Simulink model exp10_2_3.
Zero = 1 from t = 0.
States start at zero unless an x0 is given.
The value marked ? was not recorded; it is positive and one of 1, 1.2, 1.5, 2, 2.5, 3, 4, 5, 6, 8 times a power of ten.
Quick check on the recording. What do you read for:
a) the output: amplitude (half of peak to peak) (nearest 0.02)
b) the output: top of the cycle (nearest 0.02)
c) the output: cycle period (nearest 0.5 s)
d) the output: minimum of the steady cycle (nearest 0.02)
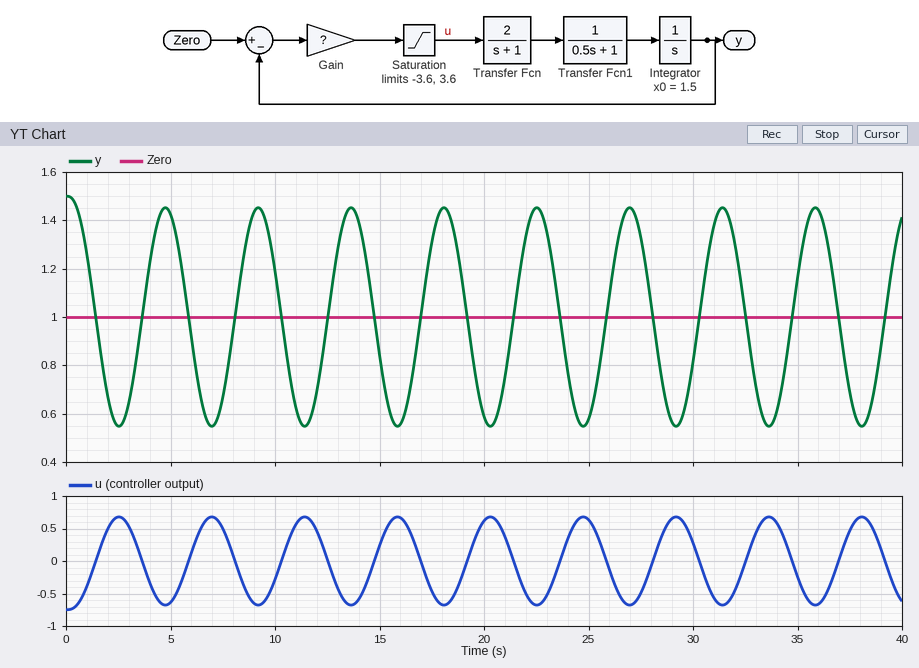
0.46
1.46
4.5 s
0.54
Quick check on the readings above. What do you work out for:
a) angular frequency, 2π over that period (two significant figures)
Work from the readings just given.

1.4 rad/s
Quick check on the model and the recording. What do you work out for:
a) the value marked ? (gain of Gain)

1.5
